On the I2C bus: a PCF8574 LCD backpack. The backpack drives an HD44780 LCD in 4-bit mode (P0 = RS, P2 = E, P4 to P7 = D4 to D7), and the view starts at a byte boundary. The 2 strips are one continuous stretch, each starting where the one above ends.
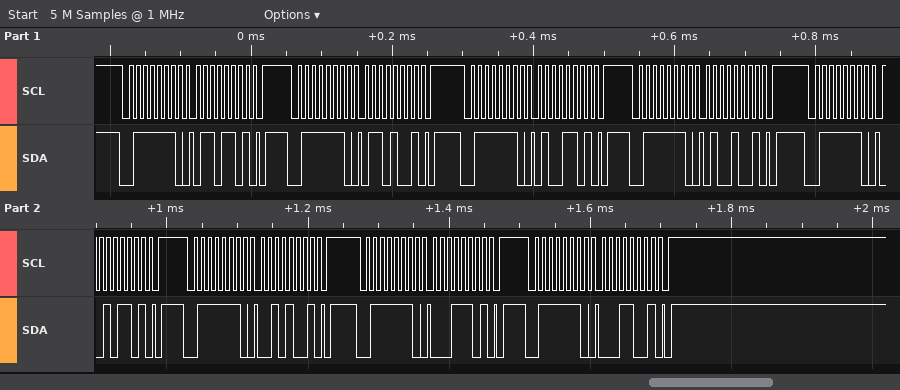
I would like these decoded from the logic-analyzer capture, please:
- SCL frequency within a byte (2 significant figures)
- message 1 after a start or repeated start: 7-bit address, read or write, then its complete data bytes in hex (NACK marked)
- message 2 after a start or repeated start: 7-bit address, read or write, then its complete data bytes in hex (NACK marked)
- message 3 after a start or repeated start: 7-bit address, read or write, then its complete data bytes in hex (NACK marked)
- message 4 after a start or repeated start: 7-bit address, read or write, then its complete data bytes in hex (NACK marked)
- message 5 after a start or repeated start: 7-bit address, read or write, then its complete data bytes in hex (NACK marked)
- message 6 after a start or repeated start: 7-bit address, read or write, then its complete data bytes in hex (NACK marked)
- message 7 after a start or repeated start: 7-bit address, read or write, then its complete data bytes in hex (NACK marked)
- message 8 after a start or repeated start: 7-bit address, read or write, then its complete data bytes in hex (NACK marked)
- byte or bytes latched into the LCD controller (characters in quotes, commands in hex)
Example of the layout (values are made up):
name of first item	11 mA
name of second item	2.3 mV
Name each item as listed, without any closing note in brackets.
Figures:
SCL frequency within a byte	100 kHz
message 1 after a start or repeated start: 7-bit address, read or write, then its complete data bytes in hex	0x3F write: 6D
message 2 after a start or repeated start: 7-bit address, read or write, then its complete data bytes in hex	0x3F write: 69
message 3 after a start or repeated start: 7-bit address, read or write, then its complete data bytes in hex	0x3F write: 4D
message 4 after a start or repeated start: 7-bit address, read or write, then its complete data bytes in hex	0x3F write: 49
message 5 after a start or repeated start: 7-bit address, read or write, then its complete data bytes in hex	0x3F write: 2D
message 6 after a start or repeated start: 7-bit address, read or write, then its complete data bytes in hex	0x3F write: 29
message 7 after a start or repeated start: 7-bit address, read or write, then its complete data bytes in hex	0x3F write: 1D
message 8 after a start or repeated start: 7-bit address, read or write, then its complete data bytes in hex	0x3F write: 19
byte or bytes latched into the LCD controller	'd' '!'
